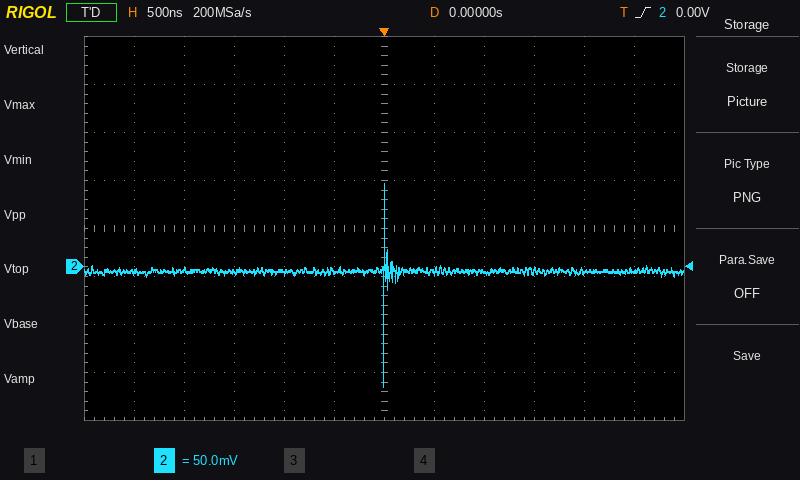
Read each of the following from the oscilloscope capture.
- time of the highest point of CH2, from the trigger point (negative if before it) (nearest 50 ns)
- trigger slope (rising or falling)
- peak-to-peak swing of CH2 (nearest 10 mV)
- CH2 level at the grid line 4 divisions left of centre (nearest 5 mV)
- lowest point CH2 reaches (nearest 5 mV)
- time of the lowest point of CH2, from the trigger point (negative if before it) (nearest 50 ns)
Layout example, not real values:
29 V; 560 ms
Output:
0 ns; rising; 210 mV; -5 mV; -125 mV; 0 ns
